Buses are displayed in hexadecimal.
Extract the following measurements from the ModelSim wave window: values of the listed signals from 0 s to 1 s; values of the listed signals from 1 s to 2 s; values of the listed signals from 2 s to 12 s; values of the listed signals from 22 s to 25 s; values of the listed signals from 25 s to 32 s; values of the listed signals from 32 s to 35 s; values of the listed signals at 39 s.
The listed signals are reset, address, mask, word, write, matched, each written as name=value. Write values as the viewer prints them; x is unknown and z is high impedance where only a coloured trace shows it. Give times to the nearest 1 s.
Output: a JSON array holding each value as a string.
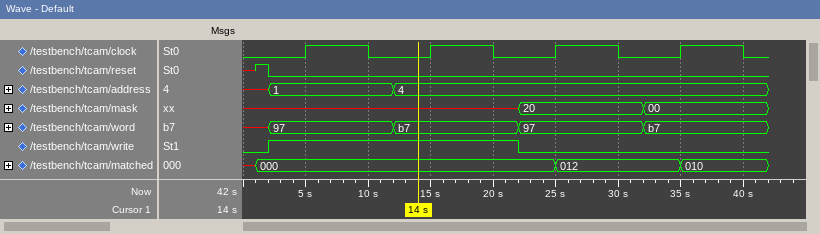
["reset=x, address=x, mask=x, word=x, write=0, matched=x", "reset=1, address=x, mask=x, word=x, write=0, matched=000", "reset=0, address=1, mask=x, word=97, write=1, matched=000", "reset=0, address=4, mask=20, word=97, write=0, matched=000", "reset=0, address=4, mask=20, word=97, write=0, matched=012", "reset=0, address=4, mask=00, word=b7, write=0, matched=012", "reset=0, address=4, mask=00, word=b7, write=0, matched=010"]
